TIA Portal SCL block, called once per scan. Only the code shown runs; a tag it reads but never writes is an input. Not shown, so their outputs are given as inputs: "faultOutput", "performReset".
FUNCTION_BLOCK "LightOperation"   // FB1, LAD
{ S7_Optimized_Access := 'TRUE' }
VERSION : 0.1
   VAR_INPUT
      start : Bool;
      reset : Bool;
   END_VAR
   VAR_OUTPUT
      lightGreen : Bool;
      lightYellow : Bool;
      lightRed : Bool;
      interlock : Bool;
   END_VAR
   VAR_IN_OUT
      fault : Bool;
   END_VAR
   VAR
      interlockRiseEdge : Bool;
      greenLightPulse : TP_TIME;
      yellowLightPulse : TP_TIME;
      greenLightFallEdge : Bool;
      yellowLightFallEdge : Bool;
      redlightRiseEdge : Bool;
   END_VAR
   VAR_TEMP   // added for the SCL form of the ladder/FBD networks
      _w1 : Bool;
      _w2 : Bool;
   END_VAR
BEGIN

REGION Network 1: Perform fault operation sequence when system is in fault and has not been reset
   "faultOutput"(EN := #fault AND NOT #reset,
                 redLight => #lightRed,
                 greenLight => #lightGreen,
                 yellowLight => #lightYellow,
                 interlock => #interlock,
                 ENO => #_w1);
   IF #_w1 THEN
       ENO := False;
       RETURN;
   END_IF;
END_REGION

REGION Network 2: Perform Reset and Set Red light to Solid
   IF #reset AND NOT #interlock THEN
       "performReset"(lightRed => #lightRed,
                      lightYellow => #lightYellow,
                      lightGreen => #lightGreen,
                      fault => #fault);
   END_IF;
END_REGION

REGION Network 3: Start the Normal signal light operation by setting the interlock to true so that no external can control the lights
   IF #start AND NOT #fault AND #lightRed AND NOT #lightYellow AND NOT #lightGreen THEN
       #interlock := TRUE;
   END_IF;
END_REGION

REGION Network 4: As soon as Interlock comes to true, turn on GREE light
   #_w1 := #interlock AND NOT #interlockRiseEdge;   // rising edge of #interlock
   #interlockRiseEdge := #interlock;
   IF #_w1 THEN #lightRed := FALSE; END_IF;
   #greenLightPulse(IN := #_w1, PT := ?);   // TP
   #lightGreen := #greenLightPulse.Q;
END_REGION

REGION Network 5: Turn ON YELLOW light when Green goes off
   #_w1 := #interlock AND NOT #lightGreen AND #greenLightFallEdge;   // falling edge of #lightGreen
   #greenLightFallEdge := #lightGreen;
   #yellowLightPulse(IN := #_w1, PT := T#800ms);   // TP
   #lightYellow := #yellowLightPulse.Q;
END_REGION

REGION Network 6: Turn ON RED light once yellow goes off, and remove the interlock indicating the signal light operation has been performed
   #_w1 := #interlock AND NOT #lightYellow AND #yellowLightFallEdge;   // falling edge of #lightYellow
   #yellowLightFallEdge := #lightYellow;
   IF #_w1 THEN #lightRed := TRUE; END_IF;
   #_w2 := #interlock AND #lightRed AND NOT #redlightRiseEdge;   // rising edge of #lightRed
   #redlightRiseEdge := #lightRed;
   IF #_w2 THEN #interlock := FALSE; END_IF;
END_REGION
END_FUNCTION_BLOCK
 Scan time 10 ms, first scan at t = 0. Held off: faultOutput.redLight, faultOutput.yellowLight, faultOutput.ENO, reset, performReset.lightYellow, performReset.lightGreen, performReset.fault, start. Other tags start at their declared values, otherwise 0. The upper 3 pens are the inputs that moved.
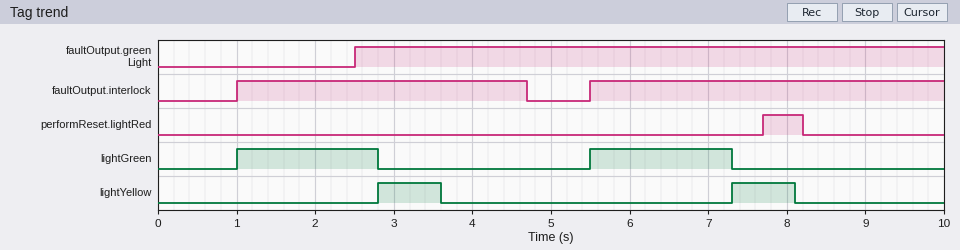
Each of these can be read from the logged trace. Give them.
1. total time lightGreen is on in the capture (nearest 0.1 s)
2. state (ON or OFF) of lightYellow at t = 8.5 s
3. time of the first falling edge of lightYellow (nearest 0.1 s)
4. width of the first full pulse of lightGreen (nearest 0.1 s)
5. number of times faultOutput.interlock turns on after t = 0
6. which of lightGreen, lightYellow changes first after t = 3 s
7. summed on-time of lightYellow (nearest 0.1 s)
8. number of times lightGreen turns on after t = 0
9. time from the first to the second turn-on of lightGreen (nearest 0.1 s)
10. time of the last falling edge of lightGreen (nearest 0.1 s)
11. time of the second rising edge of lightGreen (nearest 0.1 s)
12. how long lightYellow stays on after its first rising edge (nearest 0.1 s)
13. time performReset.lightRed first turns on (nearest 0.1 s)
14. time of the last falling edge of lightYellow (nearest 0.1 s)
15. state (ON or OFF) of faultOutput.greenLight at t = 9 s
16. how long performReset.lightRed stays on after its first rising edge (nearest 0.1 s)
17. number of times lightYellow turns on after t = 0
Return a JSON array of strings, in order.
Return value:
["3.6 s", "OFF", "3.6 s", "1.8 s", "2", "lightYellow", "1.6 s", "2", "4.5 s", "7.3 s", "5.5 s", "0.8 s", "7.7 s", "8.1 s", "ON", "0.5 s", "2"]
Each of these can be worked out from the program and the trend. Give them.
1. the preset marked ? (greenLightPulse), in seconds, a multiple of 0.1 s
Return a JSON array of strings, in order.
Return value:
["1.8 s"]
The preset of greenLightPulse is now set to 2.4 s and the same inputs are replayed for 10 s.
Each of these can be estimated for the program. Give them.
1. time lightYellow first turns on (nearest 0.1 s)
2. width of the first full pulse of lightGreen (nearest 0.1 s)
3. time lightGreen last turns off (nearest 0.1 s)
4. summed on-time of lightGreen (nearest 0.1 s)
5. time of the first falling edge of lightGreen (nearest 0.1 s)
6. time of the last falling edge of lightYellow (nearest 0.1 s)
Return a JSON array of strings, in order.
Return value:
["3.4 s", "2.4 s", "7.9 s", "4.8 s", "3.4 s", "8.7 s"]
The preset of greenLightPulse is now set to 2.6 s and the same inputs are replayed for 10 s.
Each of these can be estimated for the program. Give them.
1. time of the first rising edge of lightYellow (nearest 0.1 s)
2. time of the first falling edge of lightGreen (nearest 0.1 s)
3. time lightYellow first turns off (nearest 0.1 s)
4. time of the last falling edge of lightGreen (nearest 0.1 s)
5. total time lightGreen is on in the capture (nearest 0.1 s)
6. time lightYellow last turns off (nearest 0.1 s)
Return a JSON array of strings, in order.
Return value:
["3.6 s", "3.6 s", "4.4 s", "8.1 s", "5.2 s", "8.9 s"]
